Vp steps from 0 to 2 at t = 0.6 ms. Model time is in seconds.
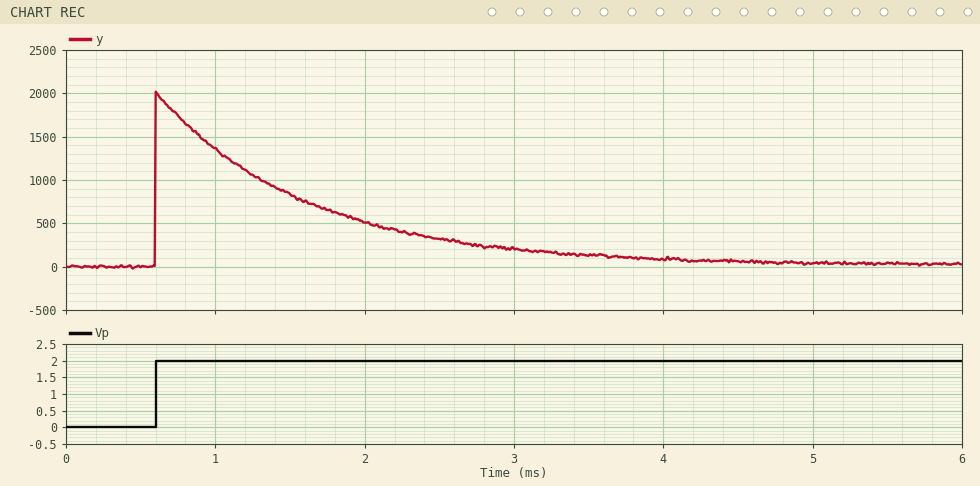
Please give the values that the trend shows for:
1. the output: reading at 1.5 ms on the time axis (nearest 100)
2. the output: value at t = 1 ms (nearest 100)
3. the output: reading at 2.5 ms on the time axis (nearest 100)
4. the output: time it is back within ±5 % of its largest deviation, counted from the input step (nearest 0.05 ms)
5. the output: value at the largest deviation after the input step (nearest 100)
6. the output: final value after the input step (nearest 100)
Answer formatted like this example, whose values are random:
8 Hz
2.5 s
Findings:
800
1400
300
3.00 ms
2000
0
